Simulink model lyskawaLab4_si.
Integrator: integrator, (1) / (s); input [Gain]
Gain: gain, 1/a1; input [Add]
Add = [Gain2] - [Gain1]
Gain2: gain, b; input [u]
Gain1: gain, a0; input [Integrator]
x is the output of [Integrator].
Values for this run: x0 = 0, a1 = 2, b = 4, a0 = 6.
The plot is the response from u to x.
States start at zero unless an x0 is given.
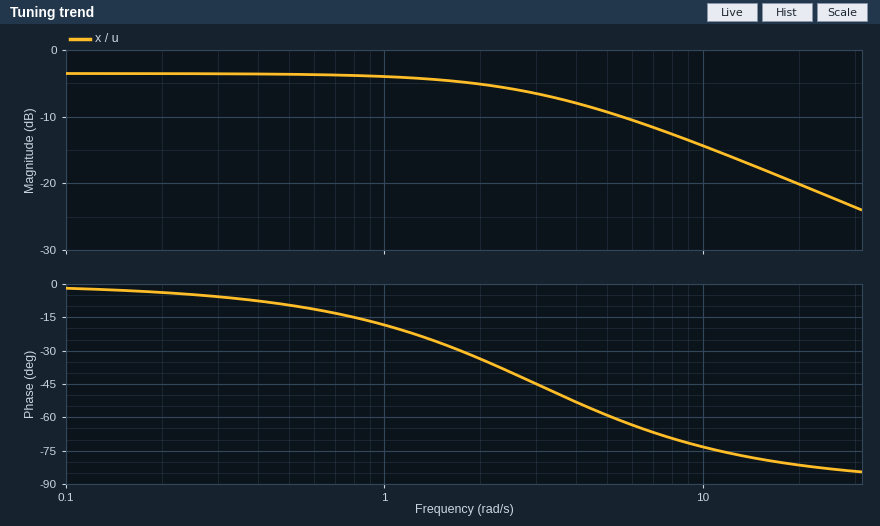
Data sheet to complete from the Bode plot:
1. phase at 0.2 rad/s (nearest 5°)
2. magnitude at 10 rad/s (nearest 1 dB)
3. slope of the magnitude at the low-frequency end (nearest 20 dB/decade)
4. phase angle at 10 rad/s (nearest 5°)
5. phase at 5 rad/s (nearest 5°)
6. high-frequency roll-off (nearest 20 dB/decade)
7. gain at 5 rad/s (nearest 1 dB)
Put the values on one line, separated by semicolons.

-5°; -14 dB; 0 dB/decade; -75°; -60°; -20 dB/decade; -9 dB
